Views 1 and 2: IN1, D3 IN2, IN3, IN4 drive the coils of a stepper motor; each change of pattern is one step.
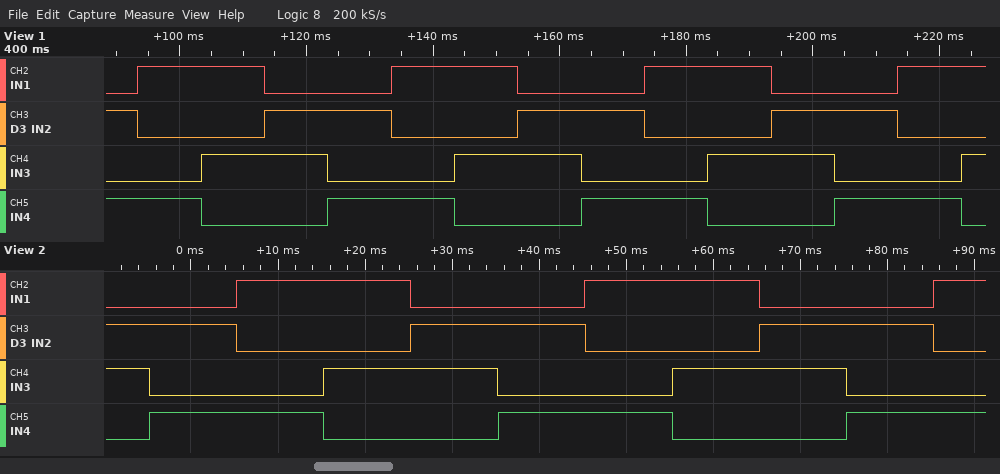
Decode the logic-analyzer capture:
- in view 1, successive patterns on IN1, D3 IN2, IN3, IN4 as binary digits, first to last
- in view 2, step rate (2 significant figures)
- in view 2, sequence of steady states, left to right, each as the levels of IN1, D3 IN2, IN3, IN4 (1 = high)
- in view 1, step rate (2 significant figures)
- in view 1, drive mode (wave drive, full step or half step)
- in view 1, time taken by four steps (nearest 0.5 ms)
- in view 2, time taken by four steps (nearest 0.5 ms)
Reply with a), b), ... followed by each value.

a) 0101 1001 1010 0110 0101 1001 1010 0110 0101 1001 1010 0110 0101 1001 1010
b) 100 steps/s
c) 0110 0101 1001 1010 0110 0101 1001 1010 0110 0101 1001
d) 100 steps/s
e) full step
f) 40.0 ms
g) 40.0 ms
